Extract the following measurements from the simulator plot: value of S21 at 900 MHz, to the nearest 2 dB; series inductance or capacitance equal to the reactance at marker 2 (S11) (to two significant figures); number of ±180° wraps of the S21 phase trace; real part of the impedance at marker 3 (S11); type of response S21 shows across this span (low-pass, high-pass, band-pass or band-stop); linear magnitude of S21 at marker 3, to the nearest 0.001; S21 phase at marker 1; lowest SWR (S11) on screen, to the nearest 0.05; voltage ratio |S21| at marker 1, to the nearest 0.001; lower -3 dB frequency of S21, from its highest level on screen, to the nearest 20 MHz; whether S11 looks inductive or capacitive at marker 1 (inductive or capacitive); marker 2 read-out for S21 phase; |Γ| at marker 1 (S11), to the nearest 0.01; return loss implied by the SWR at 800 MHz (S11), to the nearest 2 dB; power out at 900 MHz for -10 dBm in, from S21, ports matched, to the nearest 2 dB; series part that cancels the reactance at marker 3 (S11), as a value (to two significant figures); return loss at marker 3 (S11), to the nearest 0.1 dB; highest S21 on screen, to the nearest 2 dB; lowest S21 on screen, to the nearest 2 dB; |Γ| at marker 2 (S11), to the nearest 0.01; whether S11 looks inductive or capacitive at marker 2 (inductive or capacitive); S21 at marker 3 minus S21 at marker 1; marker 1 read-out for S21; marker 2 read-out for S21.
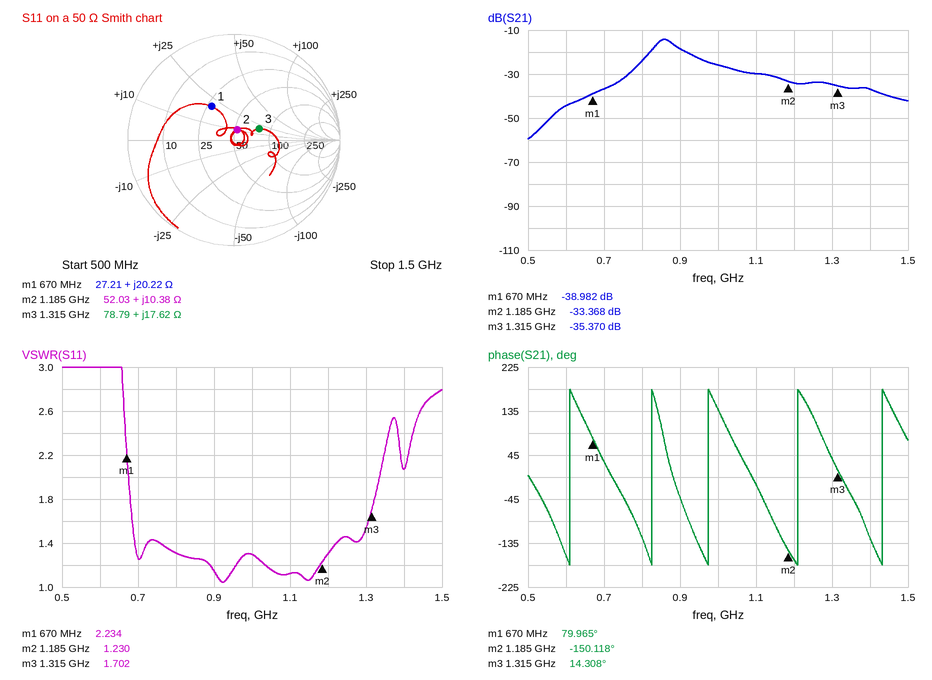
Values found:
-18 dB
1.4 nH
5
78.79 Ω
band-pass
0.017
79.965°
1.05
0.011
840 MHz
inductive
-150.118°
0.38
18 dB
-28 dBm
6.9 pF
11.7 dB
-14 dB
-60 dB
0.10
inductive
3.612 dB
-38.982 dB
-33.368 dB
